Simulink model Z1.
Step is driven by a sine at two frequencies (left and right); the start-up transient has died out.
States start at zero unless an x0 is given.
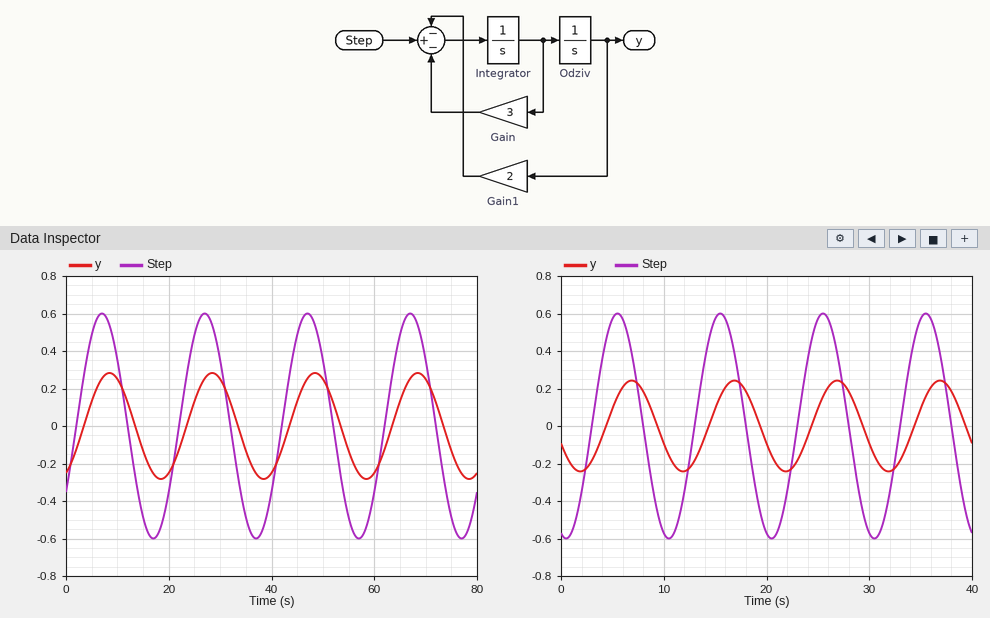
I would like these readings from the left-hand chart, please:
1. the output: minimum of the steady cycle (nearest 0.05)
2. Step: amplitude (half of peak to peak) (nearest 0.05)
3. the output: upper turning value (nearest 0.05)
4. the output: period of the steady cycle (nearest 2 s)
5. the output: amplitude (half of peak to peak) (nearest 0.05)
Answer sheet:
-0.30
0.60
0.30
20 s
0.30
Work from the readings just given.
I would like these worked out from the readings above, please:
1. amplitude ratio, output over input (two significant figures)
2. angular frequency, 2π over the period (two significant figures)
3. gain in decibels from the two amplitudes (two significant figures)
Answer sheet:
0.50
0.31 rad/s
-6.0 dB
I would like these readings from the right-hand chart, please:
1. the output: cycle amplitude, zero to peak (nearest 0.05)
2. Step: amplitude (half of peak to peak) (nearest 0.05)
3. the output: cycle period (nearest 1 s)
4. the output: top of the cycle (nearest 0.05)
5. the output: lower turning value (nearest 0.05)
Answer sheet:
0.25
0.60
10 s
0.25
-0.25
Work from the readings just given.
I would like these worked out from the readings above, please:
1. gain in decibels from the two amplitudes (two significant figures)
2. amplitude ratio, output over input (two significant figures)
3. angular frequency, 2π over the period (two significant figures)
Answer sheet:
-7.6 dB
0.42
0.63 rad/s
